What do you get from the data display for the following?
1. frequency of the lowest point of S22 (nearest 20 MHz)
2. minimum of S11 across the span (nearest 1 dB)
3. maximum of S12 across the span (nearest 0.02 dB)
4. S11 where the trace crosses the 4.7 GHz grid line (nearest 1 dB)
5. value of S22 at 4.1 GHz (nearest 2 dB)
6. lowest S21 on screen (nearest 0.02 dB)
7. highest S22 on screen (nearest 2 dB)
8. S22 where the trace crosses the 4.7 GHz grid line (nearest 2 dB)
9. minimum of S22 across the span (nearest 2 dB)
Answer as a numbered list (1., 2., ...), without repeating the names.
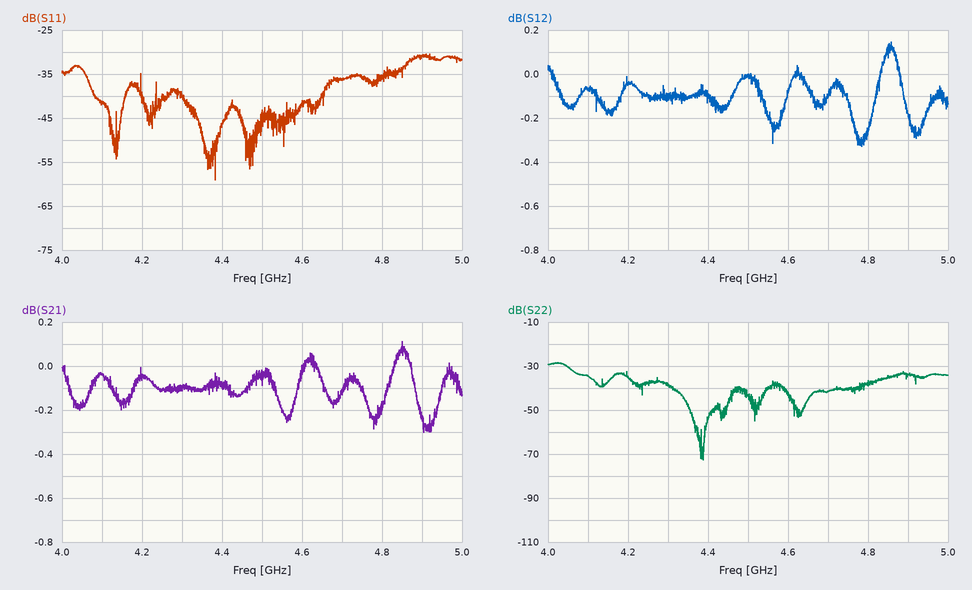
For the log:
1. 4.38 GHz
2. -59 dB
3. 0.14 dB
4. -36 dB
5. -34 dB
6. -0.30 dB
7. -28 dB
8. -42 dB
9. -72 dB
